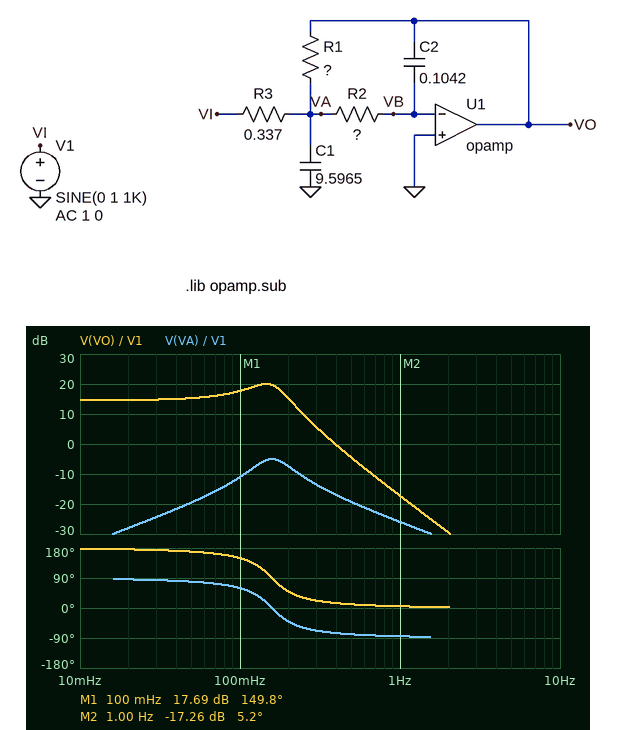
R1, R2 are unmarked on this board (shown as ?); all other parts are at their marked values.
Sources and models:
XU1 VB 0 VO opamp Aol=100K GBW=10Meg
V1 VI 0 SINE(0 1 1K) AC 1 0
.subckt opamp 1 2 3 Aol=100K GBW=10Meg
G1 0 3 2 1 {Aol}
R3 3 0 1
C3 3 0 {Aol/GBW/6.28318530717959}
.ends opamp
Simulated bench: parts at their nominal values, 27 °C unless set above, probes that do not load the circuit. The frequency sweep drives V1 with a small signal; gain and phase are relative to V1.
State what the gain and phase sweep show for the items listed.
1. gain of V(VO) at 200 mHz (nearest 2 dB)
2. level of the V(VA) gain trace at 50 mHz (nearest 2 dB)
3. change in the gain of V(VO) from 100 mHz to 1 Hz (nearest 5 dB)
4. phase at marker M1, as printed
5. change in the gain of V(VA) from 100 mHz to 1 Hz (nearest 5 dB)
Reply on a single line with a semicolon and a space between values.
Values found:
16 dB; -20 dB; -35 dB; 149.8 deg; -15 dB
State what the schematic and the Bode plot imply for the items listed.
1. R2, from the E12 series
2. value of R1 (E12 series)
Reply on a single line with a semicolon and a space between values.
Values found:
0.56 Ω; 1.8 Ω
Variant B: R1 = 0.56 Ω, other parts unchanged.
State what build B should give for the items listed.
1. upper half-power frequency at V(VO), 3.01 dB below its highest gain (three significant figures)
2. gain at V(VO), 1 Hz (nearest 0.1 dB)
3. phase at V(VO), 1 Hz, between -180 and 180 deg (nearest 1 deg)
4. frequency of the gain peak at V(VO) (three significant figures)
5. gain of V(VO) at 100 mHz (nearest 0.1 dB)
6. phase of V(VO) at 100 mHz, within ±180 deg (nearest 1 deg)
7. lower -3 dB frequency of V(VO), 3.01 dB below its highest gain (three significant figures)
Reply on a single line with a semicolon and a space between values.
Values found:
324 mHz; -16.8 dB; 7 deg; 274 mHz; 5.5 dB; 171 deg; 211 mHz
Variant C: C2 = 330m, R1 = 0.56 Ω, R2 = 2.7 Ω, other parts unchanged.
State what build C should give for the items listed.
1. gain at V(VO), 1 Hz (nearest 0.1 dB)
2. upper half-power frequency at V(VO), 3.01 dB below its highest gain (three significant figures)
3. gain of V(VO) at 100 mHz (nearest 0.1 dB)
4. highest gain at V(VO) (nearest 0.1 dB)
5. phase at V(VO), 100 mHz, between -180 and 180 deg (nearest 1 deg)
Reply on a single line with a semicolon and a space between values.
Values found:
-41.1 dB; 81.8 mHz; -0.9 dB; 4.9 dB; 61 deg
